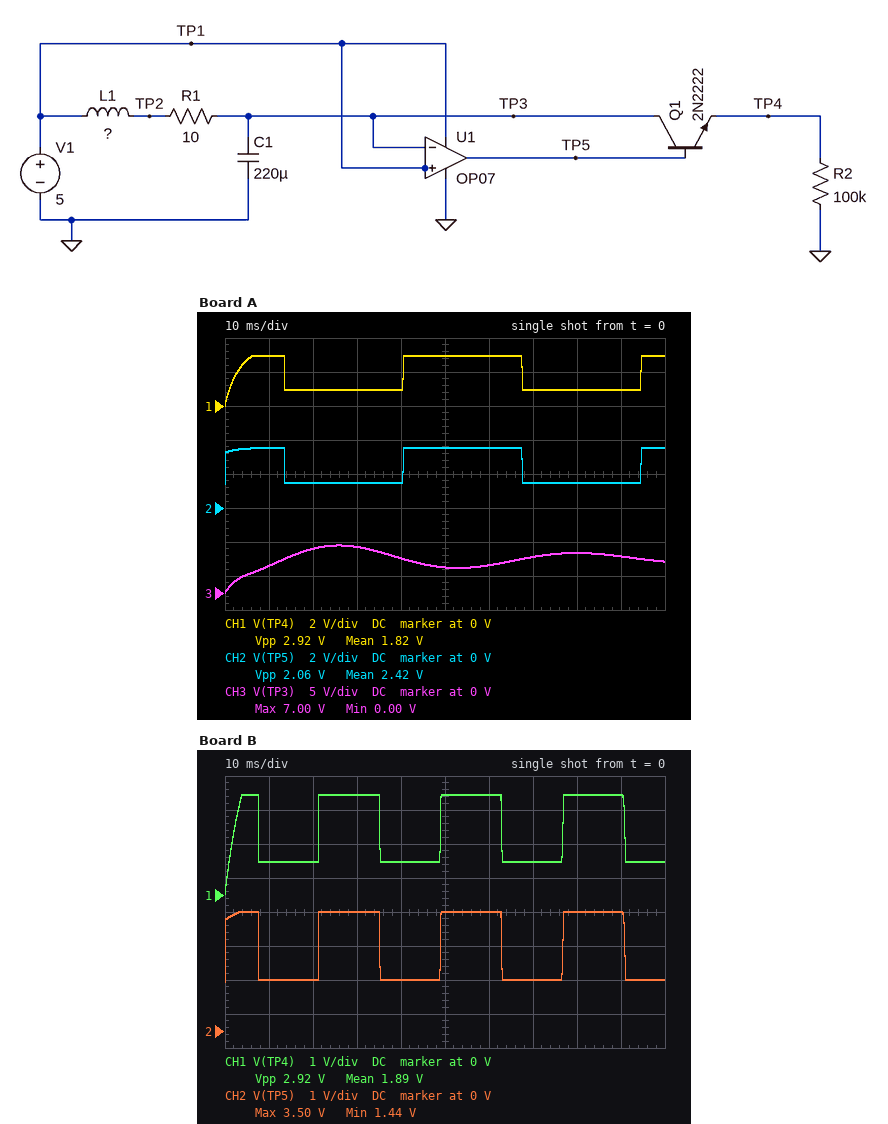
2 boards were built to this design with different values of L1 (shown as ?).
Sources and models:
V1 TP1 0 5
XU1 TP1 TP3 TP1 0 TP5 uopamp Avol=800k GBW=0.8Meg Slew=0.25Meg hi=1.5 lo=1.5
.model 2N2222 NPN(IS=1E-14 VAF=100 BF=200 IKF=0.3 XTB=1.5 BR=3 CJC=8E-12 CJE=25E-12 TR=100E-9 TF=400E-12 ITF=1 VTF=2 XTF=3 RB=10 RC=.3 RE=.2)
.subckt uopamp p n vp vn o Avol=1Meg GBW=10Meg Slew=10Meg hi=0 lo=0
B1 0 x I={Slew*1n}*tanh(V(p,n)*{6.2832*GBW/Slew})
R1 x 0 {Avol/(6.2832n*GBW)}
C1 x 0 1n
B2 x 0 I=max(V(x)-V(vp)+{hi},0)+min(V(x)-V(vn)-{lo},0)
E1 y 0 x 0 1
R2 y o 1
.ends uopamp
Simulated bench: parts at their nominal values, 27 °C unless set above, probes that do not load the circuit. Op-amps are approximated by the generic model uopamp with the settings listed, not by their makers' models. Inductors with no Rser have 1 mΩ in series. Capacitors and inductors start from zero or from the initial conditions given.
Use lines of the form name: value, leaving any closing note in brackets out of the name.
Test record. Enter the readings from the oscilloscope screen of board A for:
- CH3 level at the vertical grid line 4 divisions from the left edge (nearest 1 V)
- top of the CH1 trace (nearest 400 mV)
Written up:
CH3 level at the vertical grid line 4 divisions from the left edge: 5 V
top of the CH1 trace: 2.8 V
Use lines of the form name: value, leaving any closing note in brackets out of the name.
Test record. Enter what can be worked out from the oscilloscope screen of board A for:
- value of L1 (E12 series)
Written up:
value of L1: 330 mH
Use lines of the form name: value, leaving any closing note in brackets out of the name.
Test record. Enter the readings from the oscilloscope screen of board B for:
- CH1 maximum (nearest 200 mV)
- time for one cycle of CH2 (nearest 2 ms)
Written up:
CH1 maximum: 3.0 V
time for one cycle of CH2: 28 ms
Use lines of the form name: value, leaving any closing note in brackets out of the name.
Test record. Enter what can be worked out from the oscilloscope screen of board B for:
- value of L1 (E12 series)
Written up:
value of L1: 82 mH
